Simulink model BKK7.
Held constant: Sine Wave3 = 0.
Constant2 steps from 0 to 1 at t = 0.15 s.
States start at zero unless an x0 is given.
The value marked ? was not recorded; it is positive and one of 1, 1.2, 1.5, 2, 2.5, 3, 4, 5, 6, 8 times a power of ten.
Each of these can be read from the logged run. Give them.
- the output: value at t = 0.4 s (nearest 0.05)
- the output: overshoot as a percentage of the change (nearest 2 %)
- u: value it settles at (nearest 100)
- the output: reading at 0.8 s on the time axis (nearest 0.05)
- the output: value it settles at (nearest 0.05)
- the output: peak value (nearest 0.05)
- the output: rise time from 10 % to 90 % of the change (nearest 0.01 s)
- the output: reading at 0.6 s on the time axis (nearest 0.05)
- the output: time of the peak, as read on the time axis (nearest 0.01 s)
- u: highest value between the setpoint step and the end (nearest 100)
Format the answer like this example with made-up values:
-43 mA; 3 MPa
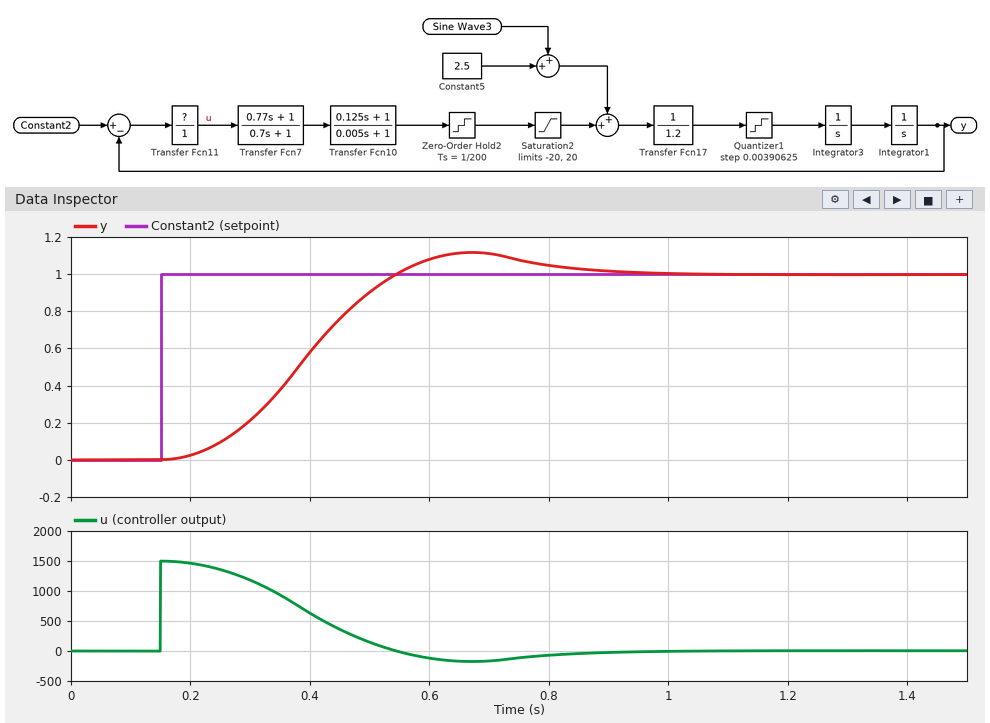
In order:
0.60; 12 %; 0; 1.05; 1.00; 1.10; 0.25 s; 1.10; 0.67 s; 1500
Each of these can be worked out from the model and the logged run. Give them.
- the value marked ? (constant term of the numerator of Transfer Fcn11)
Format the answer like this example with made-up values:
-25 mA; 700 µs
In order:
1500
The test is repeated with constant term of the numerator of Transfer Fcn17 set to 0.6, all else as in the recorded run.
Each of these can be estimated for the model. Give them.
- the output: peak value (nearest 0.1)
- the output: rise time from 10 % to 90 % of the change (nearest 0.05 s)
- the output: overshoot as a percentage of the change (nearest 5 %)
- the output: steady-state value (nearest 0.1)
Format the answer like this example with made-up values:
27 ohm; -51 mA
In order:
1.3; 0.30 s; 30 %; 1.0
